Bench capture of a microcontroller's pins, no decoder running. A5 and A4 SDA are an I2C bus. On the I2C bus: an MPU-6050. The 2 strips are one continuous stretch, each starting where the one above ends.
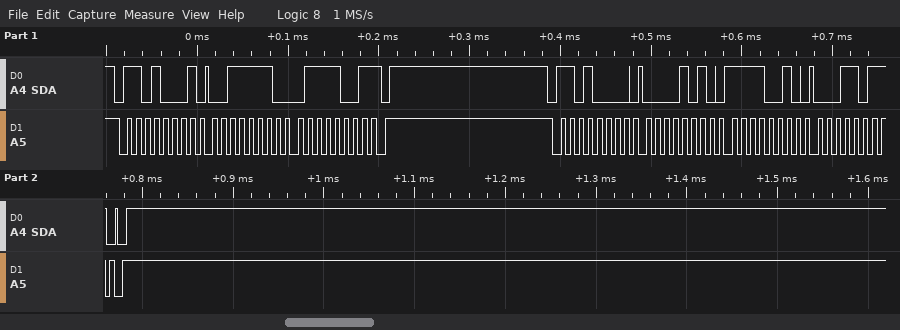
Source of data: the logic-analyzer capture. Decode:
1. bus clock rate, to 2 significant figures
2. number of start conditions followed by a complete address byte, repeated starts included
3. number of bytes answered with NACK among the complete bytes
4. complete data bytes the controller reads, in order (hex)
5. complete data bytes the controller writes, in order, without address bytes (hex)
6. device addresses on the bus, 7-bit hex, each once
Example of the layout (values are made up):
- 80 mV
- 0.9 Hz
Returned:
- 100 kHz
- 2
- 1
- 3E 79
- 0A F2 1B
- 0x68
